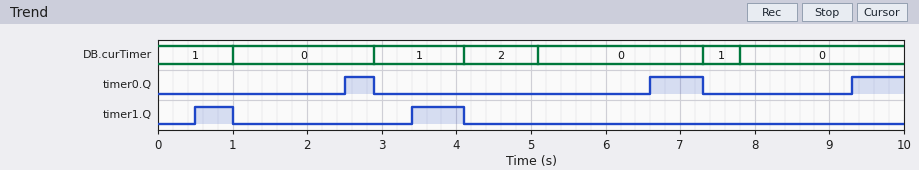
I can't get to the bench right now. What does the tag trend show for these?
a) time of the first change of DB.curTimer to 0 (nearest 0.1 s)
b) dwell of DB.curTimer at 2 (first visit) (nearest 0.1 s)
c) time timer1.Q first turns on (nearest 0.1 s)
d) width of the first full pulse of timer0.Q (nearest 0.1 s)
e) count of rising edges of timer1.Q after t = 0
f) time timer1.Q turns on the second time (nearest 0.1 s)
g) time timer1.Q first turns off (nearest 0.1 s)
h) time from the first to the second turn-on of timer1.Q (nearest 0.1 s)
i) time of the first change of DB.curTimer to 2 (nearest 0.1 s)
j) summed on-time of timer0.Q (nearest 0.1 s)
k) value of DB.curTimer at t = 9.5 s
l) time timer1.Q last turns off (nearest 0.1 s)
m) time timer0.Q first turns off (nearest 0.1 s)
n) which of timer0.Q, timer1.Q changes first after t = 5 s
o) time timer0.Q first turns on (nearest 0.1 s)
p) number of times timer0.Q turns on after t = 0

1.0 s
1.0 s
0.5 s
0.4 s
2
3.4 s
1.0 s
2.9 s
4.1 s
1.8 s
0
4.1 s
2.9 s
timer0.Q
2.5 s
3
